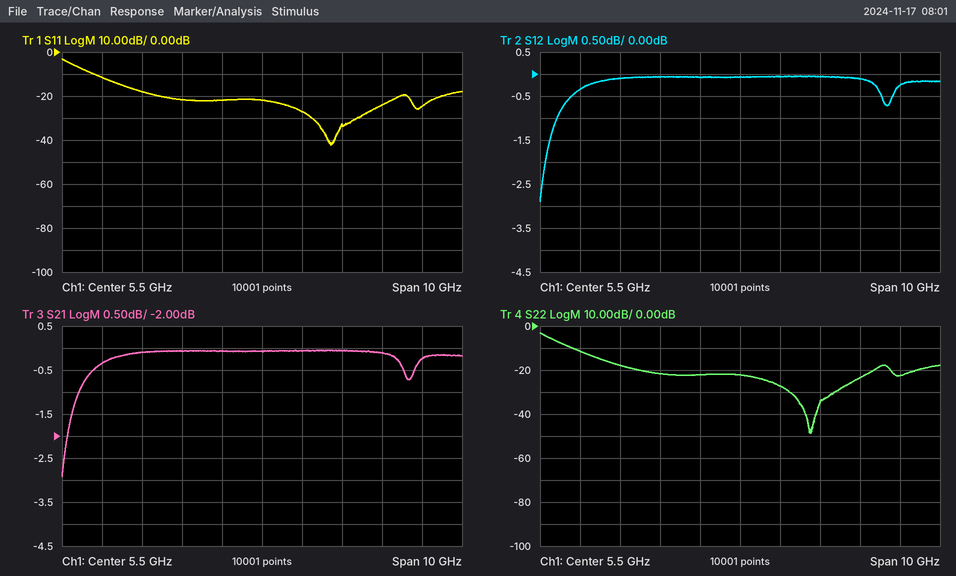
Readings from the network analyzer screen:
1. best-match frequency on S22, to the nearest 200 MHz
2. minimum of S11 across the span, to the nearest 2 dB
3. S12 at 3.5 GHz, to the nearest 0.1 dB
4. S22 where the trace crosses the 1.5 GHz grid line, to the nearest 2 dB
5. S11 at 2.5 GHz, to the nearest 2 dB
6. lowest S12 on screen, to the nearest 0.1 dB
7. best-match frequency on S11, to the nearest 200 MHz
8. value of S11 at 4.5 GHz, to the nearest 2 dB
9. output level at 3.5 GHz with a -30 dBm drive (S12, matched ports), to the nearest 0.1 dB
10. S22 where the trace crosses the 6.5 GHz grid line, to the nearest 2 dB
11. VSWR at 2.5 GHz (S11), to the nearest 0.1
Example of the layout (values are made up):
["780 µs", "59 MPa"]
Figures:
["7.2 GHz", "-42 dB", "-0.1 dB", "-12 dB", "-18 dB", "-2.9 dB", "7.2 GHz", "-22 dB", "-30.1 dBm", "-28 dB", "1.3"]
